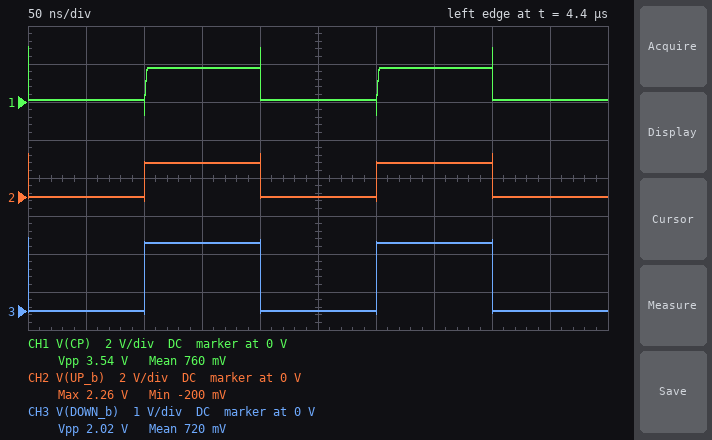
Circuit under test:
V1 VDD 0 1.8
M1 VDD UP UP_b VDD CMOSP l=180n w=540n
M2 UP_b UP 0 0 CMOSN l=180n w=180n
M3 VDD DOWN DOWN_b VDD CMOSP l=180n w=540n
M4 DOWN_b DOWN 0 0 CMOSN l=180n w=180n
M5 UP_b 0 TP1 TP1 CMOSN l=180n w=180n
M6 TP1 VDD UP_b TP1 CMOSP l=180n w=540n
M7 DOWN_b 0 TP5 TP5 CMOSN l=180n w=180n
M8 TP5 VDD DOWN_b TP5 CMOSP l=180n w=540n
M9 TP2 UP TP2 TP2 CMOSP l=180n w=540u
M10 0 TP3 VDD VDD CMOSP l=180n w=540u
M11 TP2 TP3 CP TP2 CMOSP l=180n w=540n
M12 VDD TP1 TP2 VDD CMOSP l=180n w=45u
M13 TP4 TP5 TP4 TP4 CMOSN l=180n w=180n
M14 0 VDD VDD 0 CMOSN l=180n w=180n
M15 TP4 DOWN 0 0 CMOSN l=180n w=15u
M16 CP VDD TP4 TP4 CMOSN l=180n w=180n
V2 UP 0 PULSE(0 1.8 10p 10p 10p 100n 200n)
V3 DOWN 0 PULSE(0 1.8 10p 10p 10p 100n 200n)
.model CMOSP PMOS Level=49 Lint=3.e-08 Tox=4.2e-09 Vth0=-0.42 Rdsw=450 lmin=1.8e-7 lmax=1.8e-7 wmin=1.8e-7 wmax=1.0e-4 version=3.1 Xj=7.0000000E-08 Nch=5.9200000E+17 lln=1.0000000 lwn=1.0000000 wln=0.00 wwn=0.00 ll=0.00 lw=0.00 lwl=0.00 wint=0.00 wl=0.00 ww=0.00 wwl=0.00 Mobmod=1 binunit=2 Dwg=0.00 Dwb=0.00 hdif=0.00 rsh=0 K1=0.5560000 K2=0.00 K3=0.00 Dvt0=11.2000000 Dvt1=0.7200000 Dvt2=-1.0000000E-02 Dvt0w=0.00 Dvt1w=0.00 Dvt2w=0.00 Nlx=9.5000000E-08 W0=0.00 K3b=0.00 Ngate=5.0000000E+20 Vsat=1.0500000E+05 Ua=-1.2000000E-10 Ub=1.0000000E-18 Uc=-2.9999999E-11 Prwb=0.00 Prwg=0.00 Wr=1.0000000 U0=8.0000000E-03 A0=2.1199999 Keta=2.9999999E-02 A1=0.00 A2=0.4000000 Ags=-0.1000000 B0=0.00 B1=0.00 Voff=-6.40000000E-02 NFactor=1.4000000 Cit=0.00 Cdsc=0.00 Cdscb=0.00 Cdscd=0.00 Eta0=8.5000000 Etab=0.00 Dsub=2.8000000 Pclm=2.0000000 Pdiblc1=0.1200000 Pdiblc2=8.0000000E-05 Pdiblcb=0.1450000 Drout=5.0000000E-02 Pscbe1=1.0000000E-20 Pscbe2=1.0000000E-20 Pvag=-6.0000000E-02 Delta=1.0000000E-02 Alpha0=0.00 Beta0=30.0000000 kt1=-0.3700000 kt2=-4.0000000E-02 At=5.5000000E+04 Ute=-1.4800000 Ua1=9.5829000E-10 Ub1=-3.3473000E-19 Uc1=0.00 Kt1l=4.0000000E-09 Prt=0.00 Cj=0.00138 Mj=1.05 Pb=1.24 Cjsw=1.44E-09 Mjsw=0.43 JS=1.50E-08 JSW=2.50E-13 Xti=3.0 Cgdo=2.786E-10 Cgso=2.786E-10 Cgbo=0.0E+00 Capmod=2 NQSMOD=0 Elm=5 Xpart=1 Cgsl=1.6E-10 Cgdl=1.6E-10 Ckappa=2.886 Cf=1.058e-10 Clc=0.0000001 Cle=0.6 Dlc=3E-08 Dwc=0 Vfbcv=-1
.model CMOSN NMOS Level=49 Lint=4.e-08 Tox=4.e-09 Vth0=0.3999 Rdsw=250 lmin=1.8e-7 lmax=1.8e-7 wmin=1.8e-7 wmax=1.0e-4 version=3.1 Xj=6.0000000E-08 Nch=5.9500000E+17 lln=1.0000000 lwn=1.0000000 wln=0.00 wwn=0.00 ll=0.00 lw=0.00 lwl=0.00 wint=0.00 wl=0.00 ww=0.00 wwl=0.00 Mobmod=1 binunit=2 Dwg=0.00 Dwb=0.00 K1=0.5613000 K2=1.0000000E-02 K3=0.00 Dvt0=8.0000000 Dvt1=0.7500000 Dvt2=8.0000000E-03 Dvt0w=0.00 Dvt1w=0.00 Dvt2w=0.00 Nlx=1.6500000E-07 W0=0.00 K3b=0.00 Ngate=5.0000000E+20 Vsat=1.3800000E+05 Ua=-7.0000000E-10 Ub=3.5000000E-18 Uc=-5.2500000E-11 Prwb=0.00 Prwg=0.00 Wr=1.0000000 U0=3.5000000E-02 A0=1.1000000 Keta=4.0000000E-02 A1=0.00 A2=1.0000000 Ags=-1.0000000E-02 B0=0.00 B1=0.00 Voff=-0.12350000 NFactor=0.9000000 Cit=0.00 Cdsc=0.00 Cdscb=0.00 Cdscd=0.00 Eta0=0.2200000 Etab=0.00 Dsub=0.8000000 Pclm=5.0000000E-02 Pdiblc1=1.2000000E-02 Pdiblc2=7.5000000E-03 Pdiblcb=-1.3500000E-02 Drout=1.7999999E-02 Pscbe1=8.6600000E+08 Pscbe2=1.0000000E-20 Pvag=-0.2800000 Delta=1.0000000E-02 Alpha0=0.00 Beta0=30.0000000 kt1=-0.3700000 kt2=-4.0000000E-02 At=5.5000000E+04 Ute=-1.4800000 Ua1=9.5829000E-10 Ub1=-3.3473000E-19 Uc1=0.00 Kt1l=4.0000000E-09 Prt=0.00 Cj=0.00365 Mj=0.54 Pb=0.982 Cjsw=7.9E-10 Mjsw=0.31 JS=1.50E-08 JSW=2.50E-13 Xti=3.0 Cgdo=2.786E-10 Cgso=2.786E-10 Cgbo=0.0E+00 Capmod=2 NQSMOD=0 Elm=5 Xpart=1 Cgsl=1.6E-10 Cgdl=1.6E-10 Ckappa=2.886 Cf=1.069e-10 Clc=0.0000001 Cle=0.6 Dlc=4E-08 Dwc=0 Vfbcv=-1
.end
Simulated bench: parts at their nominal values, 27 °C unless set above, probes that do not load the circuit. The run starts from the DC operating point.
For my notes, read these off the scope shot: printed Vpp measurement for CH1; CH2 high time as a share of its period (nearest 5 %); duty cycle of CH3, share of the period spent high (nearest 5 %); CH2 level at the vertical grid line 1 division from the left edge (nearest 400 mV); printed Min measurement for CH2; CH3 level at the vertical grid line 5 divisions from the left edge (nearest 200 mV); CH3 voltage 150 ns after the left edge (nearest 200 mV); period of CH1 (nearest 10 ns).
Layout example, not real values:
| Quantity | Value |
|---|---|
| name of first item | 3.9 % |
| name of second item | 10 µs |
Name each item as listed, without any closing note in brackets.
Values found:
| Quantity | Value |
|---|---|
| printed Vpp measurement for CH1 | 3.54 V |
| CH2 high time as a share of its period | 50 % |
| duty cycle of CH3, share of the period spent high | 50 % |
| CH2 level at the vertical grid line 1 division from the left edge | 0 V |
| printed Min measurement for CH2 | -200 mV |
| CH3 level at the vertical grid line 5 divisions from the left edge | 0 V |
| CH3 voltage 150 ns after the left edge | 1.8 V |
| period of CH1 | 200 ns |
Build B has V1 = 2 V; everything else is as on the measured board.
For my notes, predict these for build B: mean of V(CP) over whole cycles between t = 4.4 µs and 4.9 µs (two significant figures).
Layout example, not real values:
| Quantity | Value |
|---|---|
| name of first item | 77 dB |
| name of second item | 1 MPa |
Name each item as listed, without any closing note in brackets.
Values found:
| Quantity | Value |
|---|---|
| mean of V(CP) over whole cycles between t = 4.4 µs and 4.9 µs | 1.0 V |
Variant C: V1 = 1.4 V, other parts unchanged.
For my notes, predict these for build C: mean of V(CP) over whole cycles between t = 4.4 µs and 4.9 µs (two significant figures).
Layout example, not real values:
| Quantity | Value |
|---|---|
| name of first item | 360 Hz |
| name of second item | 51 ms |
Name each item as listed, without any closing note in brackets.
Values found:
| Quantity | Value |
|---|---|
| mean of V(CP) over whole cycles between t = 4.4 µs and 4.9 µs | 700 mV |
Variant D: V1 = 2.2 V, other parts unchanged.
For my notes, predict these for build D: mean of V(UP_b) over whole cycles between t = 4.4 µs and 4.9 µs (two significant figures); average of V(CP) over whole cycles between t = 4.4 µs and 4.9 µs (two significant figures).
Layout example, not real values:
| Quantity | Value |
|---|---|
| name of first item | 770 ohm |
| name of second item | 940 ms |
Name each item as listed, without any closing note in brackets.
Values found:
| Quantity | Value |
|---|---|
| mean of V(UP_b) over whole cycles between t = 4.4 µs and 4.9 µs | 1.1 V |
| average of V(CP) over whole cycles between t = 4.4 µs and 4.9 µs | 1.2 V |
